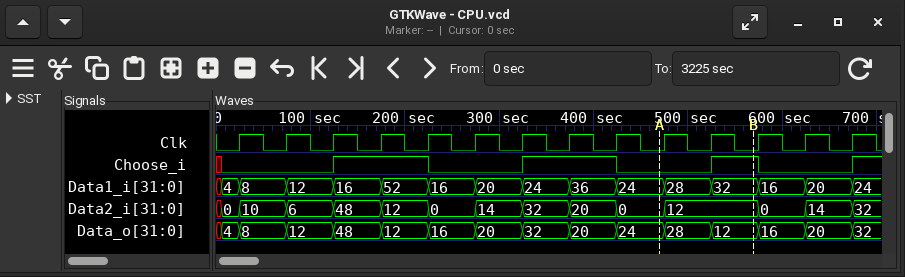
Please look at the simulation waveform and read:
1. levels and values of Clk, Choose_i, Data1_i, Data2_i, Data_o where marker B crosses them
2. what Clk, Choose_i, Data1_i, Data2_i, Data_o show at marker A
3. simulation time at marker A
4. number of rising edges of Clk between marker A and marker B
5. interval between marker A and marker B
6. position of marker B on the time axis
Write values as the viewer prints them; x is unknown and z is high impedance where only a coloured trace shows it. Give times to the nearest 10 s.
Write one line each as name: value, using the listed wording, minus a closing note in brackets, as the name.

levels and values of Clk, Choose_i, Data1_i, Data2_i, Data_o where marker B crosses them: Clk=0, Choose_i=1, Data1_i=32, Data2_i=12, Data_o=12
what Clk, Choose_i, Data1_i, Data2_i, Data_o show at marker A: Clk=0, Choose_i=0, Data1_i=24, Data2_i=0, Data_o=24
simulation time at marker A: 470 s
number of rising edges of Clk between marker A and marker B: 2
interval between marker A and marker B: 100 s
position of marker B on the time axis: 570 s
